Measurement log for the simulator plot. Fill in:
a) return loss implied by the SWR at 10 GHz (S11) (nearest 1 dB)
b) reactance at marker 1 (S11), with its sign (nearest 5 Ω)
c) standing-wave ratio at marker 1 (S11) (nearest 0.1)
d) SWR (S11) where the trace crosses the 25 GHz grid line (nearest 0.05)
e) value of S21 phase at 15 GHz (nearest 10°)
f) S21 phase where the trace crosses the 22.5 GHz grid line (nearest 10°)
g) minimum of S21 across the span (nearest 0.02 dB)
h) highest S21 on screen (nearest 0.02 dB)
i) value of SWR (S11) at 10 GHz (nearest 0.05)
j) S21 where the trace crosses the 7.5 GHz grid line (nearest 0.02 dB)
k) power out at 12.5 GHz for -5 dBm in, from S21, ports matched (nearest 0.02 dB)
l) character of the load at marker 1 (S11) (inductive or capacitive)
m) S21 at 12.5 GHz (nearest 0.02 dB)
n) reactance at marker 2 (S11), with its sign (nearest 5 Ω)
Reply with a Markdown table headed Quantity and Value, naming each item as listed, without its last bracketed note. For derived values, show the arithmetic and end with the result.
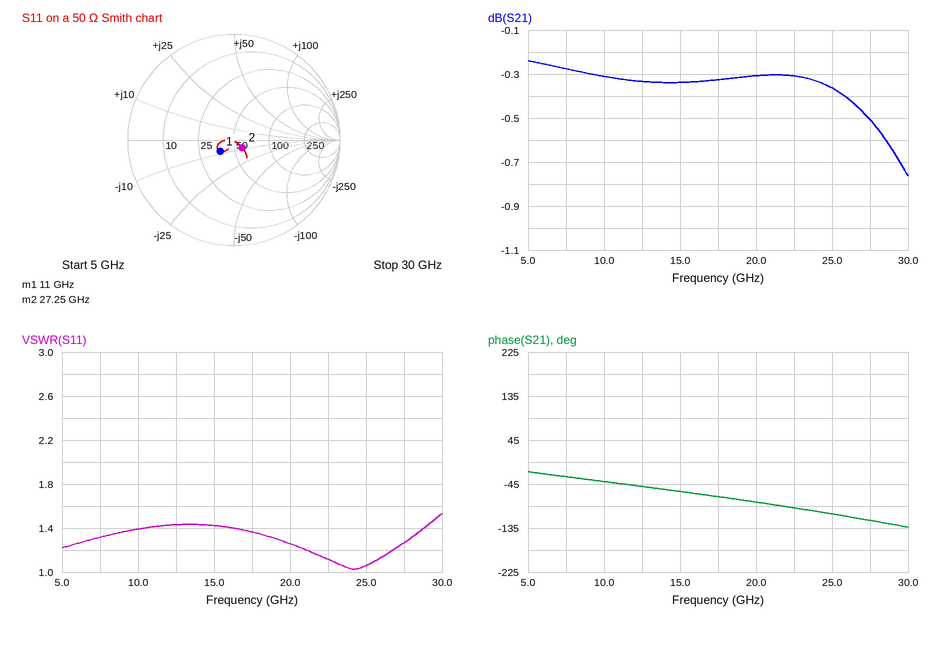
| Quantity | Value |
|---|---|
| return loss implied by the SWR at 10 GHz (S11) | −20 log10((1.4 − 1)/(1.4 + 1)) ≈ 16 dB |
| reactance at marker 1 (S11), with its sign | -10 Ω |
| standing-wave ratio at marker 1 (S11) | 1.4 |
| SWR (S11) where the trace crosses the 25 GHz grid line | 1.05 |
| value of S21 phase at 15 GHz | -60° |
| S21 phase where the trace crosses the 22.5 GHz grid line | -90° |
| minimum of S21 across the span | -0.76 dB |
| highest S21 on screen | -0.24 dB |
| value of SWR (S11) at 10 GHz | 1.40 |
| S21 where the trace crosses the 7.5 GHz grid line | -0.28 dB |
| power out at 12.5 GHz for -5 dBm in, from S21, ports matched | -5 dBm + (-0.34 dB) = -5.34 dBm |
| character of the load at marker 1 (S11) | capacitive |
| S21 at 12.5 GHz | -0.34 dB |
| reactance at marker 2 (S11), with its sign | -10 Ω |
